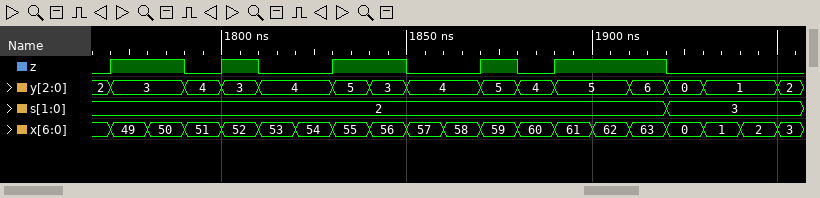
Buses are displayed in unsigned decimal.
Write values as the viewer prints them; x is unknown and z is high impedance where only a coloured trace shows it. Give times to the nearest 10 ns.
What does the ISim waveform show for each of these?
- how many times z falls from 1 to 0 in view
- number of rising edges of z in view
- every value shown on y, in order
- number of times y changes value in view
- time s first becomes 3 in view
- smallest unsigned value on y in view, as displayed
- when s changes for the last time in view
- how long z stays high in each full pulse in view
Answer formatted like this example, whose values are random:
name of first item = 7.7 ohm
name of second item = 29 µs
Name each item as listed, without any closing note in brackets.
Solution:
how many times z falls from 1 to 0 in view = 5
number of rising edges of z in view = 5
every value shown on y, in order = 2, 3, 4, 3, 4, 5, 3, 4, 5, 4, 5, 6, 0, 1, 2
number of times y changes value in view = 14
time s first becomes 3 in view = 1920 ns
smallest unsigned value on y in view, as displayed = 0
when s changes for the last time in view = 1920 ns
how long z stays high in each full pulse in view = 20 ns, 10 ns, 20 ns, 10 ns, 30 ns
